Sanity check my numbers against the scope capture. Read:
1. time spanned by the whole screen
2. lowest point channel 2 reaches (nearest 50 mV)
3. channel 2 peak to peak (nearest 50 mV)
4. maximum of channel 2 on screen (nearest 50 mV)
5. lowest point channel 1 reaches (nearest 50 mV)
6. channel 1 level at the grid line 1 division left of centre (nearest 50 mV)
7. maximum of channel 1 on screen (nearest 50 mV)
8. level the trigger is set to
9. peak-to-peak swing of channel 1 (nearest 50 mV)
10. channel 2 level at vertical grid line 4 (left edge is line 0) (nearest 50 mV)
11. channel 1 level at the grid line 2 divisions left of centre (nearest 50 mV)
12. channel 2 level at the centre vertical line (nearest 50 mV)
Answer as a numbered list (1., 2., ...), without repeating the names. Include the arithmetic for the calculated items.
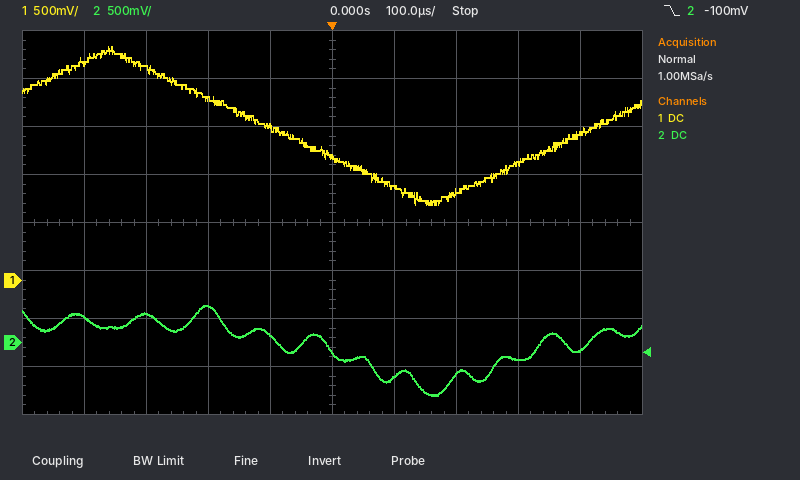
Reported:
1. 1 ms
2. -550 mV
3. 400 mV − (-550 mV) = 950 mV
4. 400 mV
5. 800 mV
6. 1.60 V
7. 2.45 V
8. -100 mV
9. 2.45 V − (800 mV) = 1.65 V
10. 100 mV
11. 1.90 V
12. -100 mV
